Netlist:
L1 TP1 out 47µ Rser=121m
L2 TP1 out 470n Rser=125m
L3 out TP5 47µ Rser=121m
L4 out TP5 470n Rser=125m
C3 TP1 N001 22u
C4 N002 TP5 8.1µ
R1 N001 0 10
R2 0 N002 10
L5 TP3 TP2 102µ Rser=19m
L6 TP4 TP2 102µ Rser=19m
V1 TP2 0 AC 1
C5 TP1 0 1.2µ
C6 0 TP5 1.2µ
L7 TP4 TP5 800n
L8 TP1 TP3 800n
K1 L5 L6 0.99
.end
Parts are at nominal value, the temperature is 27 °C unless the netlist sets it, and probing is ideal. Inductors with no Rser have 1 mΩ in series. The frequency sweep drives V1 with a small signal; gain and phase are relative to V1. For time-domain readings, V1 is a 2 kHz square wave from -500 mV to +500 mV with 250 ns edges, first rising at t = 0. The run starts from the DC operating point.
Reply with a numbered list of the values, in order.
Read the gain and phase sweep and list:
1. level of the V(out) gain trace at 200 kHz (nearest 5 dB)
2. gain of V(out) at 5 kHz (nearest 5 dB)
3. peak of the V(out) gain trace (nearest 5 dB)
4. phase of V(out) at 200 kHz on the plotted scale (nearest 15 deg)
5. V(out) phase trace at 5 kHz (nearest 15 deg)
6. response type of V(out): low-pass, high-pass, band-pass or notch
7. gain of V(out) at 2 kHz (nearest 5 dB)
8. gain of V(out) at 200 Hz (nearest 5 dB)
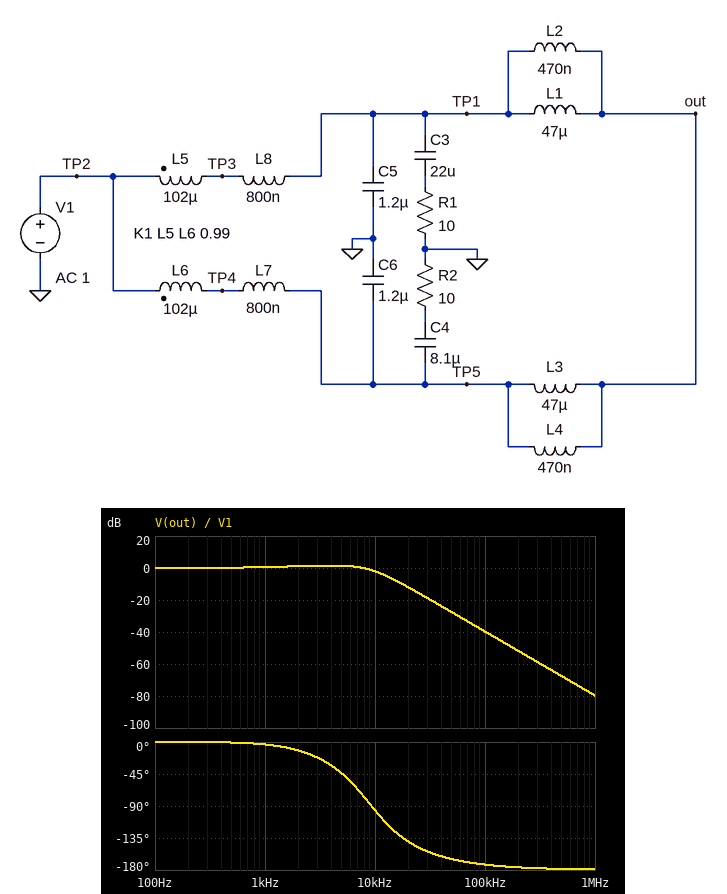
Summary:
1. -50 dB
2. 0 dB
3. 0 dB
4. -180 deg
5. -45 deg
6. low-pass
7. 0 dB
8. 0 dB
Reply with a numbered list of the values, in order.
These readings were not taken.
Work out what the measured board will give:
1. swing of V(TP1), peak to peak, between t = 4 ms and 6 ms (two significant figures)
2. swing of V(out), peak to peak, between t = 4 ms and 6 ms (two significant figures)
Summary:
1. 1.4 V
2. 1.4 V
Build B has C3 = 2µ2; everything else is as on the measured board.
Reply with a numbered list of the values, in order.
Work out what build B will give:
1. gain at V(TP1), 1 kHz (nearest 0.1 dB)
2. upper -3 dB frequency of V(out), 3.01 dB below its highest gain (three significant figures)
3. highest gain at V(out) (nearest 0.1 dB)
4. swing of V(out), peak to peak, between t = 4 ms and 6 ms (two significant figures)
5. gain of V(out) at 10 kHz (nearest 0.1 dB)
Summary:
1. 0.4 dB
2. 8.69 kHz
3. 4.2 dB
4. 1.8 V
5. -0.9 dB
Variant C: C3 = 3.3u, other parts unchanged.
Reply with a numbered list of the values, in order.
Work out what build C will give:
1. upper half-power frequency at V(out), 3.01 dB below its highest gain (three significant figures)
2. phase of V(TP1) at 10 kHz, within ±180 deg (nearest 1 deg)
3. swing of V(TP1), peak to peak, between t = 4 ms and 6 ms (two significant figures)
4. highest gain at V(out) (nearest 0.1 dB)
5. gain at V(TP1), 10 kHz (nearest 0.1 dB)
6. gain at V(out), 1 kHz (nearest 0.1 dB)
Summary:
1. 8.53 kHz
2. -106 deg
3. 1.7 V
4. 3.6 dB
5. -1.5 dB
6. 0.4 dB
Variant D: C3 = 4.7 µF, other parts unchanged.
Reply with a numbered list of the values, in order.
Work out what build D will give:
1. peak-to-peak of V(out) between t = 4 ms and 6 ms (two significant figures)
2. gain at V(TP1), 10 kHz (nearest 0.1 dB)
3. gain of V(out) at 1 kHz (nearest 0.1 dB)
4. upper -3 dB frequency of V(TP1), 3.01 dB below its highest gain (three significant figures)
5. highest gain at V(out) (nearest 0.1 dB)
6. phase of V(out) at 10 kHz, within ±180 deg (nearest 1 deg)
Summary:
1. 1.6 V
2. -1.8 dB
3. 0.5 dB
4. 8.57 kHz
5. 3.0 dB
6. -103 deg
